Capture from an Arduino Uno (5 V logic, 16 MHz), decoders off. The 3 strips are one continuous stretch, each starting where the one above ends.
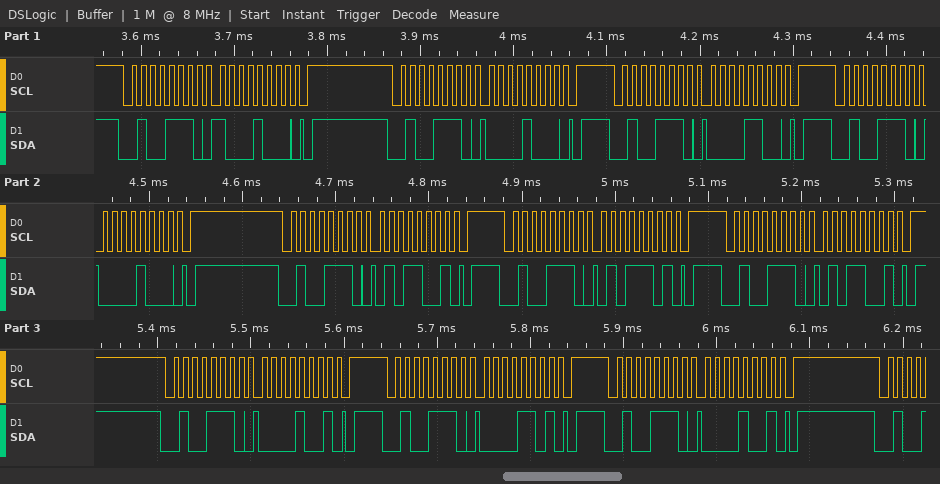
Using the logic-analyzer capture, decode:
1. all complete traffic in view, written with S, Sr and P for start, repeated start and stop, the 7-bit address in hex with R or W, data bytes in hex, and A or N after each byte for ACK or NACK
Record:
S 27W A 88 A P S 27W A 08 A P S 27W A 0C A P S 27W A 08 A P S 27W A 59 A P S 27W A 5D A P S 27W A 59 A P S 27W A 09 A P S 27W A 0D A P S 27W A 09 A P
